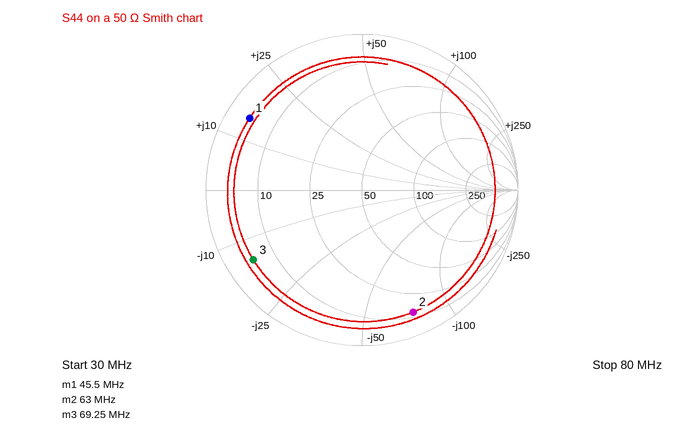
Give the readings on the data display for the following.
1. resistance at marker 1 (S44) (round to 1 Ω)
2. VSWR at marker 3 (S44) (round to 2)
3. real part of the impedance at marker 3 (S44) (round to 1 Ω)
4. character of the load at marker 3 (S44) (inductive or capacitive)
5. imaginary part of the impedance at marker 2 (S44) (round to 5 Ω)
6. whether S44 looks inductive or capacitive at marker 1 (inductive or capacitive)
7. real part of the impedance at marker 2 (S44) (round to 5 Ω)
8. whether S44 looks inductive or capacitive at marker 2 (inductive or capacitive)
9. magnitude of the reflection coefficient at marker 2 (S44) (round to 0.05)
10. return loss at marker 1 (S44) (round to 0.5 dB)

4 Ω
10
5 Ω
capacitive
-75 Ω
inductive
15 Ω
capacitive
0.85
1.5 dB
